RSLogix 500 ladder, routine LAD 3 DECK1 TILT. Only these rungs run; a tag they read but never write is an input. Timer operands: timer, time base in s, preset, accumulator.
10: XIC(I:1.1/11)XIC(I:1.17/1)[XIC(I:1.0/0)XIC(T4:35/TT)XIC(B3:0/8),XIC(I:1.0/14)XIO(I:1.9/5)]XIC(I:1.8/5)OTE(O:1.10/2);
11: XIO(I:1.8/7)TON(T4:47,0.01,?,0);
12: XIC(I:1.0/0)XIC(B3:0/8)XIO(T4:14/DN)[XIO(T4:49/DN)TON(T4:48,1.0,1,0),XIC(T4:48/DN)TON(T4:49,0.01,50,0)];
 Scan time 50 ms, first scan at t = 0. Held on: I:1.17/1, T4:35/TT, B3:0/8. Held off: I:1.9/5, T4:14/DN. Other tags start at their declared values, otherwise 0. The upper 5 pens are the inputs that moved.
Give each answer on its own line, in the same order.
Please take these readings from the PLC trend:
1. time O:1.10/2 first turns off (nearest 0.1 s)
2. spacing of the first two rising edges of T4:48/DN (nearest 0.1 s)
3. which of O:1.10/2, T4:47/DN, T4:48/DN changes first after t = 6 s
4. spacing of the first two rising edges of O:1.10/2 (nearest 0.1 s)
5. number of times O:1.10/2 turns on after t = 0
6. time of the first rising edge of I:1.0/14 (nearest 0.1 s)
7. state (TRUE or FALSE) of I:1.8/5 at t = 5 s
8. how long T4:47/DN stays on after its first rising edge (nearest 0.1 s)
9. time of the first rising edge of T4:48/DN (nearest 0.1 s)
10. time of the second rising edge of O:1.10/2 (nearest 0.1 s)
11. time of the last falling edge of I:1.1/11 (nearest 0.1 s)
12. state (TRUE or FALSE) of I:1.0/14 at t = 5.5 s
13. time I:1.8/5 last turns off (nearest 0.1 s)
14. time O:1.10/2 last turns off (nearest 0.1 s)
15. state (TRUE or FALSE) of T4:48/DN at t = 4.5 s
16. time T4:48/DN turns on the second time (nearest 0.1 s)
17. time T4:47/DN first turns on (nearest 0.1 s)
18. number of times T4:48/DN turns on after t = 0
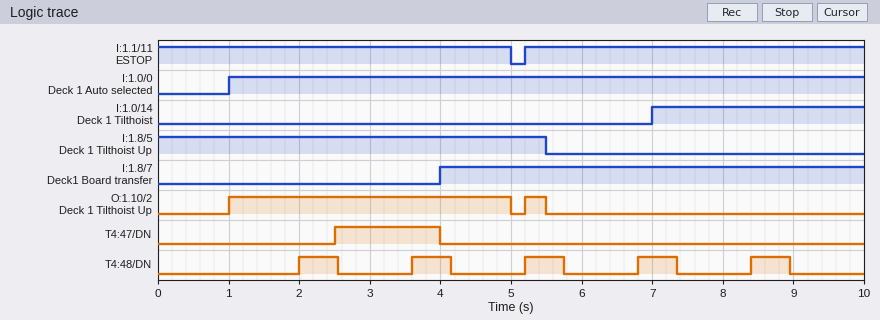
5.0 s
1.6 s
T4:48/DN
4.2 s
2
7.0 s
TRUE
1.5 s
2.0 s
5.2 s
5.0 s
FALSE
5.5 s
5.5 s
FALSE
3.6 s
2.5 s
5
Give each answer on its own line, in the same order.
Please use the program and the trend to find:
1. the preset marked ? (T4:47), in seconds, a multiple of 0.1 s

2.5 s
